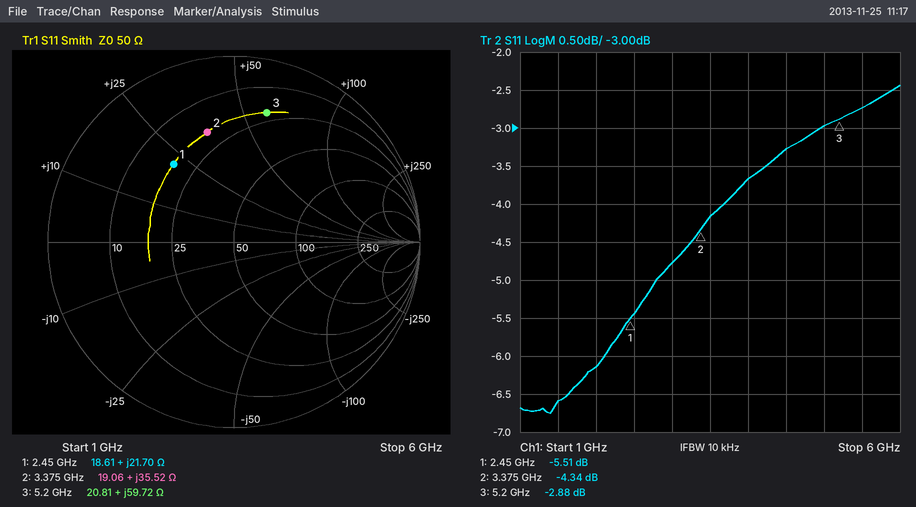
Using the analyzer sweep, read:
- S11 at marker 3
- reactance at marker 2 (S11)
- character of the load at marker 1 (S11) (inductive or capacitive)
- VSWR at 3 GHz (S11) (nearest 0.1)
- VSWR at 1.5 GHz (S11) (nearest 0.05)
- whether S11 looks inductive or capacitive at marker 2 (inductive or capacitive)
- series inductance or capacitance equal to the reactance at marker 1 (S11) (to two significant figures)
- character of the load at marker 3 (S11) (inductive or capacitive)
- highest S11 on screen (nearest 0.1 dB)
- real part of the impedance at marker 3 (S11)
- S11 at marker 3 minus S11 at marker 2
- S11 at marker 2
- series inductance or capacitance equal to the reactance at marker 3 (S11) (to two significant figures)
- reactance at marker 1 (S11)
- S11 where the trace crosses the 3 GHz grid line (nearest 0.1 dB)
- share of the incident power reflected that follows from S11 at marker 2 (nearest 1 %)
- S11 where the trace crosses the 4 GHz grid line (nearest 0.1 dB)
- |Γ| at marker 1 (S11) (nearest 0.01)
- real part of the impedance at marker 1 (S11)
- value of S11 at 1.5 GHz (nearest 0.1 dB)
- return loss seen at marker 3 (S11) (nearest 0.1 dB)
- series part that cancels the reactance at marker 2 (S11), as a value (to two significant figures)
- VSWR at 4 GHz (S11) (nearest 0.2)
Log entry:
-2.88 dB
+35.52 Ω
inductive
3.7
2.75
inductive
1.4 nH
inductive
-2.4 dB
20.81 Ω
1.46 dB
-4.34 dB
1.8 nH
+21.70 Ω
-4.8 dB
37 %
-3.7 dB
0.53
18.61 Ω
-6.6 dB
2.9 dB
1.3 pF
4.8
